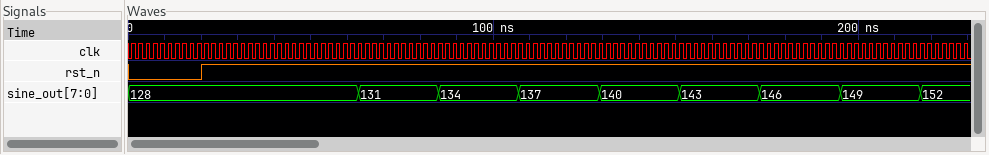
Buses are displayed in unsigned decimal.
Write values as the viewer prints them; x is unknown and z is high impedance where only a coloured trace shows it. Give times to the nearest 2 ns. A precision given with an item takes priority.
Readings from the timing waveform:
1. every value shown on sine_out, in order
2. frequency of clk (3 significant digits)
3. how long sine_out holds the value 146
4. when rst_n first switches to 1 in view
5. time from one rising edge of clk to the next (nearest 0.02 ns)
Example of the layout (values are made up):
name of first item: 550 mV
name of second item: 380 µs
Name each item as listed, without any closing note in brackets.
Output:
every value shown on sine_out, in order: 128, 131, 134, 137, 140, 143, 146, 149, 152
frequency of clk: 500 MHz
how long sine_out holds the value 146: 22 ns
when rst_n first switches to 1 in view: 20 ns
time from one rising edge of clk to the next: 2 ns
